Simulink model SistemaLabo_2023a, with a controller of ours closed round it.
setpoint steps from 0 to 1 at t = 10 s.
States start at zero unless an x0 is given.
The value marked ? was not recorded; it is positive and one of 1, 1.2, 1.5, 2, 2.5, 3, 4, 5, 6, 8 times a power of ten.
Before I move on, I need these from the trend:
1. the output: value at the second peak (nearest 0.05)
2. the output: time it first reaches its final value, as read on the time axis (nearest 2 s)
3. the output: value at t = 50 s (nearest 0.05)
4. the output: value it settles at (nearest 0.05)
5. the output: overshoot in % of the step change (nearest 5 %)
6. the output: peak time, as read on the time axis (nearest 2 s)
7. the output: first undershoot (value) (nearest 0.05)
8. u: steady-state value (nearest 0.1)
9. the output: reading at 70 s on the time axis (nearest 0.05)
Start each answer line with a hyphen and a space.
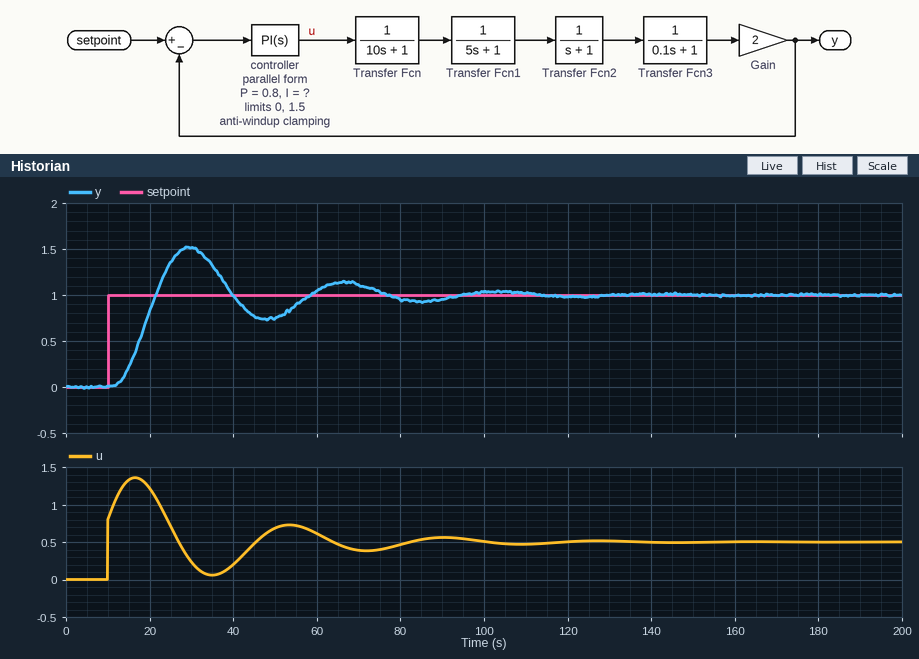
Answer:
- 1.15
- 22 s
- 0.75
- 1.00
- 50 %
- 30 s
- 0.75
- 0.5
- 1.10
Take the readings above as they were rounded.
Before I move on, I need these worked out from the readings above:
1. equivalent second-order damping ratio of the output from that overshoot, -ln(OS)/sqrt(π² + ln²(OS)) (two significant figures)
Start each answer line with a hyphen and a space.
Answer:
- 0.22
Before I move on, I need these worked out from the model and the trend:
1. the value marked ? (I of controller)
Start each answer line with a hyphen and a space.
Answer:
- 0.15
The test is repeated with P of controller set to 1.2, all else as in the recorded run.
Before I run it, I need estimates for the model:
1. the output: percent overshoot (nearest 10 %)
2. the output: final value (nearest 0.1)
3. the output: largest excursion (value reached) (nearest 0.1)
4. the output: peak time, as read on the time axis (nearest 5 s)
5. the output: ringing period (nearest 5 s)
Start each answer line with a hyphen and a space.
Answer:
- 40 %
- 1.0
- 1.4
- 25 s
- 30 s
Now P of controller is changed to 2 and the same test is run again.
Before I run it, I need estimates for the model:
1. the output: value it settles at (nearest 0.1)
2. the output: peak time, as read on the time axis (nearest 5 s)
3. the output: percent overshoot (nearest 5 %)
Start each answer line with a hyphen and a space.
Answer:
- 1.0
- 25 s
- 15 %
